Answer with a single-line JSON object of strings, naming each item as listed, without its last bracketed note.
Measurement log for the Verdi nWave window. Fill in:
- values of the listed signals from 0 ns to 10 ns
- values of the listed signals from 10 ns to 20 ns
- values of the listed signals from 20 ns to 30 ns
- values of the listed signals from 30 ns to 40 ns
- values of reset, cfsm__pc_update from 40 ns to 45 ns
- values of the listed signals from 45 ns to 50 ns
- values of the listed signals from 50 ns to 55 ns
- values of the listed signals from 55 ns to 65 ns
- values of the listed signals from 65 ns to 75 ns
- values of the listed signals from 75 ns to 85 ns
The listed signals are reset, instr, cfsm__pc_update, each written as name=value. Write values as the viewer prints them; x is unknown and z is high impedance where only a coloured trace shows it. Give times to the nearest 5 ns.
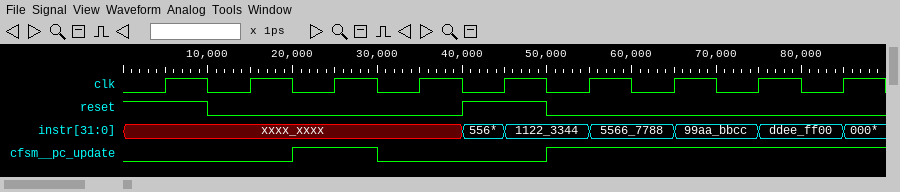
{"values of the listed signals from 0 ns to 10 ns": "reset=1, instr=xxxx_xxxx, cfsm__pc_update=0", "values of the listed signals from 10 ns to 20 ns": "reset=0, instr=xxxx_xxxx, cfsm__pc_update=0", "values of the listed signals from 20 ns to 30 ns": "reset=0, instr=xxxx_xxxx, cfsm__pc_update=1", "values of the listed signals from 30 ns to 40 ns": "reset=0, instr=xxxx_xxxx, cfsm__pc_update=0", "values of reset, cfsm__pc_update from 40 ns to 45 ns": "reset=1, cfsm__pc_update=0", "values of the listed signals from 45 ns to 50 ns": "reset=1, instr=1122_3344, cfsm__pc_update=0", "values of the listed signals from 50 ns to 55 ns": "reset=0, instr=1122_3344, cfsm__pc_update=1", "values of the listed signals from 55 ns to 65 ns": "reset=0, instr=5566_7788, cfsm__pc_update=1", "values of the listed signals from 65 ns to 75 ns": "reset=0, instr=99aa_bbcc, cfsm__pc_update=1", "values of the listed signals from 75 ns to 85 ns": "reset=0, instr=ddee_ff00, cfsm__pc_update=1"}
